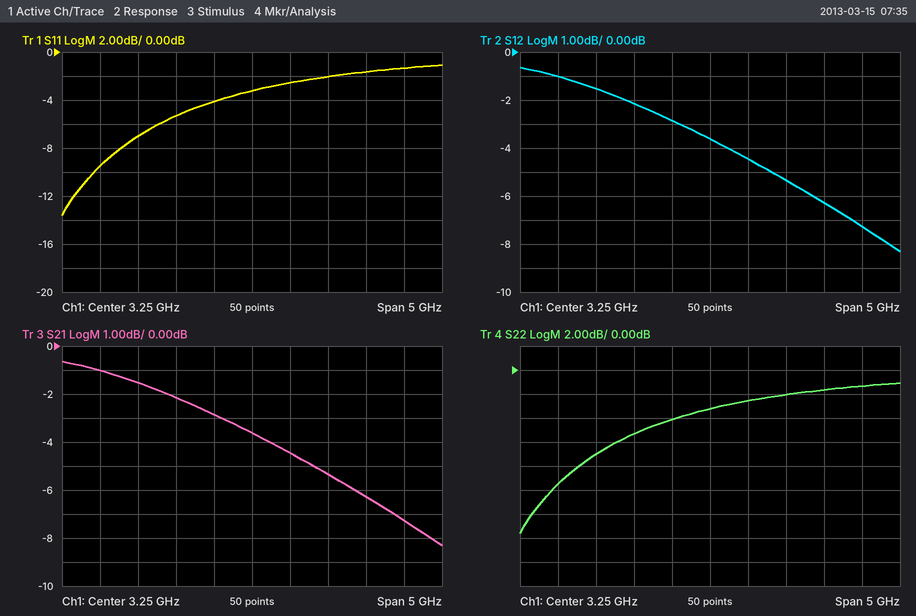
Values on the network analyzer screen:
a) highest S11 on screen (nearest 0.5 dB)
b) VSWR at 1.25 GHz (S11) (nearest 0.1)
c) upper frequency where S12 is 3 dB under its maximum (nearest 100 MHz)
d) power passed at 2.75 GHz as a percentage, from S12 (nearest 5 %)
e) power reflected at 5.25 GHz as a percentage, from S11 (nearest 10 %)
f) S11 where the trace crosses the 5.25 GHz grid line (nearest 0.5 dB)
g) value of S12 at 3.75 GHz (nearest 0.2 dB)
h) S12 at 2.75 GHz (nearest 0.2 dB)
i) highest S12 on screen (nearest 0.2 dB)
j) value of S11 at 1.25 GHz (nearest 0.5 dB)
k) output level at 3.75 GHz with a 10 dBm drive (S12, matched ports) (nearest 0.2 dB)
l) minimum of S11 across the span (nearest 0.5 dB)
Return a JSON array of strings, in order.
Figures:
["-1.0 dB", "2.0", "3.3 GHz", "50 %", "70 %", "-1.5 dB", "-4.4 dB", "-2.8 dB", "-0.6 dB", "-9.5 dB", "5.6 dBm", "-13.5 dB"]
